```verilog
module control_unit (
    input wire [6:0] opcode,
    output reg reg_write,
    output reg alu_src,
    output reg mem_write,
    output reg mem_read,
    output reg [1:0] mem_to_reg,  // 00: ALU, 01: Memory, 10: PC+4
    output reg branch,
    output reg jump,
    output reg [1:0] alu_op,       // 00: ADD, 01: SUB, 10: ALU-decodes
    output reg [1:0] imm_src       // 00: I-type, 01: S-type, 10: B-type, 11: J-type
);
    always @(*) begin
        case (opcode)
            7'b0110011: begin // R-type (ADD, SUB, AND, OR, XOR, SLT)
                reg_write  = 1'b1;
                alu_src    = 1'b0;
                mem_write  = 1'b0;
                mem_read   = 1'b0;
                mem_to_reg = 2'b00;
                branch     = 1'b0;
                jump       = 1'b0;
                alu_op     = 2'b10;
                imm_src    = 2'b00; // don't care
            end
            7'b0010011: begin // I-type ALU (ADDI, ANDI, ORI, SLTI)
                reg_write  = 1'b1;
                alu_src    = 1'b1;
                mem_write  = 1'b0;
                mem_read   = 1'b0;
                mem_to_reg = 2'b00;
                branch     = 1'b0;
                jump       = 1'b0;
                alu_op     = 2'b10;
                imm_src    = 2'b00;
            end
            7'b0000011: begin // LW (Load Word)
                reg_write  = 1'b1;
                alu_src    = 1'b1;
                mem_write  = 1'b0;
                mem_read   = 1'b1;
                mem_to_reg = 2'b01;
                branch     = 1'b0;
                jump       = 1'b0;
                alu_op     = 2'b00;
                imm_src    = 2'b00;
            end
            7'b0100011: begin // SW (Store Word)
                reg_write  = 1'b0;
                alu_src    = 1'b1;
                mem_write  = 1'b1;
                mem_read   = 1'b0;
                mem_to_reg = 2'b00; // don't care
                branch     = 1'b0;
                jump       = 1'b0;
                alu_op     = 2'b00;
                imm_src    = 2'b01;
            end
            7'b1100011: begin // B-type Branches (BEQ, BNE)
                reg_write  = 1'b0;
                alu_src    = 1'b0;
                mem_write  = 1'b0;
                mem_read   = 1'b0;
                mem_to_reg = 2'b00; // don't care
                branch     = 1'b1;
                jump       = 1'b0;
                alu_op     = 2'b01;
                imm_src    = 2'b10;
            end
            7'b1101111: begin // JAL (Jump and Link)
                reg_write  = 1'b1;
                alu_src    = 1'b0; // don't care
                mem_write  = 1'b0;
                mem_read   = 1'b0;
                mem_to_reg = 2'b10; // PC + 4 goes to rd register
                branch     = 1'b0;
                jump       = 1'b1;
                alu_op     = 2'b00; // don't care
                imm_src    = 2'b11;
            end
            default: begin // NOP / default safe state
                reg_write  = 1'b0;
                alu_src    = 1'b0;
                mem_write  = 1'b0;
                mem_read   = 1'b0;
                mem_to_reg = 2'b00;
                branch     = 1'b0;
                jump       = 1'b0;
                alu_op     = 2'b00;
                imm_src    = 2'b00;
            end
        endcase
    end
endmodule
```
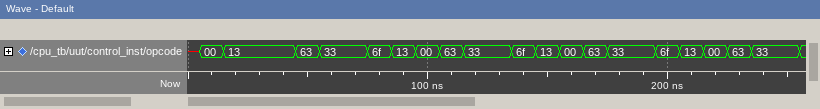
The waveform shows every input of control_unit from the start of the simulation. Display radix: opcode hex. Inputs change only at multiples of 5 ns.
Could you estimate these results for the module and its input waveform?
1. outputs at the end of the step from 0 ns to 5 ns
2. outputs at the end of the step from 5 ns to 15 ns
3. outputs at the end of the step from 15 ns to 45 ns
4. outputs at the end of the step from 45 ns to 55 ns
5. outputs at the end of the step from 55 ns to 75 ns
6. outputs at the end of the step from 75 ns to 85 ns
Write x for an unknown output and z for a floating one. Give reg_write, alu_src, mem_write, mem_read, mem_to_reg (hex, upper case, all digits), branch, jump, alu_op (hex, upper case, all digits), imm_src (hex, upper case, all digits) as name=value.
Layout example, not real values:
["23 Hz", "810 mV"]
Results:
["reg_write=x, alu_src=x, mem_write=x, mem_read=x, mem_to_reg=x, branch=x, jump=x, alu_op=x, imm_src=x", "reg_write=0, alu_src=0, mem_write=0, mem_read=0, mem_to_reg=0, branch=0, jump=0, alu_op=0, imm_src=0", "reg_write=1, alu_src=1, mem_write=0, mem_read=0, mem_to_reg=0, branch=0, jump=0, alu_op=2, imm_src=0", "reg_write=0, alu_src=0, mem_write=0, mem_read=0, mem_to_reg=0, branch=1, jump=0, alu_op=1, imm_src=2", "reg_write=1, alu_src=0, mem_write=0, mem_read=0, mem_to_reg=0, branch=0, jump=0, alu_op=2, imm_src=0", "reg_write=1, alu_src=0, mem_write=0, mem_read=0, mem_to_reg=2, branch=0, jump=1, alu_op=0, imm_src=3"]
